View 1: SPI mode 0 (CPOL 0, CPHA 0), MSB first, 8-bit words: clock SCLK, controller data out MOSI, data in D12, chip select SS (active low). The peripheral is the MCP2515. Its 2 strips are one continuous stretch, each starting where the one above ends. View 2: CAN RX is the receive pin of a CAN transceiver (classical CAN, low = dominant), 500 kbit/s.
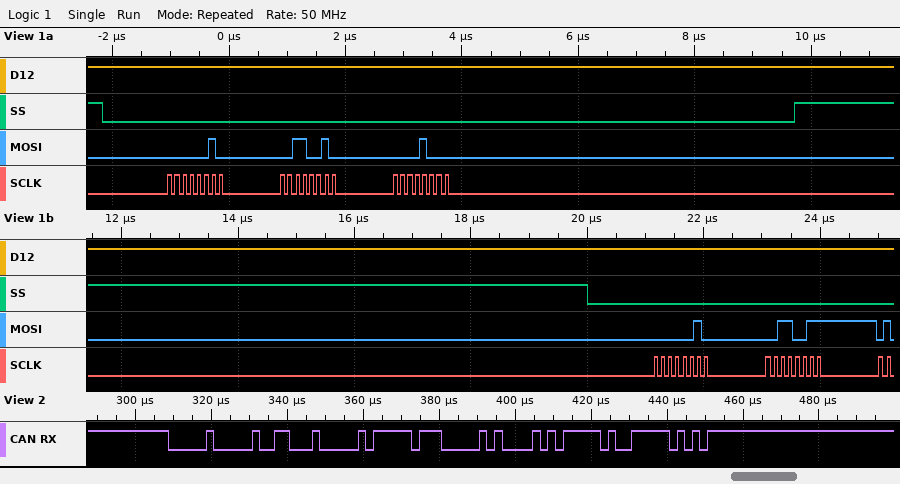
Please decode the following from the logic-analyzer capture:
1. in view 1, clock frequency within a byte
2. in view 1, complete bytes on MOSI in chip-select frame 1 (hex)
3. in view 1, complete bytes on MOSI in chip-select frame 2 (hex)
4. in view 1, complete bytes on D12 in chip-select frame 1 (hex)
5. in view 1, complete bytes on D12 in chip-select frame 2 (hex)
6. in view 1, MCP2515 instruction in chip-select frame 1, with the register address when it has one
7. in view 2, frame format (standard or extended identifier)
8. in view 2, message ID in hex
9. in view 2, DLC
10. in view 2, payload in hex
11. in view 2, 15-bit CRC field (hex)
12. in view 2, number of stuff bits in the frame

8 MHz
02 32 08
02 33
FF FF FF
FF FF
WRITE 0x32
extended
0x000040FF
1
0A
0x7E7E
7
